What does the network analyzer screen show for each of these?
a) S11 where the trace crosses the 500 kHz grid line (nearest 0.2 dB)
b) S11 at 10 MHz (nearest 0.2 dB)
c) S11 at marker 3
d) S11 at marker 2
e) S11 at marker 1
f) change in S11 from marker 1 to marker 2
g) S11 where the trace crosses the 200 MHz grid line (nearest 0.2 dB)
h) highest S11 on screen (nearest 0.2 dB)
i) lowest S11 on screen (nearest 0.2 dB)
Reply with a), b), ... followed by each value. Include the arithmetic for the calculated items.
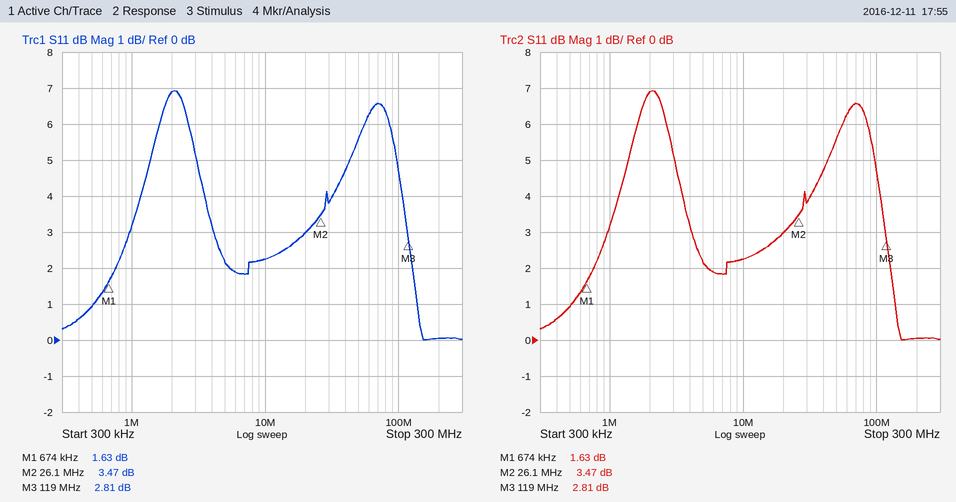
a) 1.0 dB
b) 2.2 dB
c) 2.81 dB
d) 3.47 dB
e) 1.63 dB
f) 3.47 − (1.63) = 1.84 dB
g) 0.0 dB
h) 7.0 dB
i) 0.0 dB
